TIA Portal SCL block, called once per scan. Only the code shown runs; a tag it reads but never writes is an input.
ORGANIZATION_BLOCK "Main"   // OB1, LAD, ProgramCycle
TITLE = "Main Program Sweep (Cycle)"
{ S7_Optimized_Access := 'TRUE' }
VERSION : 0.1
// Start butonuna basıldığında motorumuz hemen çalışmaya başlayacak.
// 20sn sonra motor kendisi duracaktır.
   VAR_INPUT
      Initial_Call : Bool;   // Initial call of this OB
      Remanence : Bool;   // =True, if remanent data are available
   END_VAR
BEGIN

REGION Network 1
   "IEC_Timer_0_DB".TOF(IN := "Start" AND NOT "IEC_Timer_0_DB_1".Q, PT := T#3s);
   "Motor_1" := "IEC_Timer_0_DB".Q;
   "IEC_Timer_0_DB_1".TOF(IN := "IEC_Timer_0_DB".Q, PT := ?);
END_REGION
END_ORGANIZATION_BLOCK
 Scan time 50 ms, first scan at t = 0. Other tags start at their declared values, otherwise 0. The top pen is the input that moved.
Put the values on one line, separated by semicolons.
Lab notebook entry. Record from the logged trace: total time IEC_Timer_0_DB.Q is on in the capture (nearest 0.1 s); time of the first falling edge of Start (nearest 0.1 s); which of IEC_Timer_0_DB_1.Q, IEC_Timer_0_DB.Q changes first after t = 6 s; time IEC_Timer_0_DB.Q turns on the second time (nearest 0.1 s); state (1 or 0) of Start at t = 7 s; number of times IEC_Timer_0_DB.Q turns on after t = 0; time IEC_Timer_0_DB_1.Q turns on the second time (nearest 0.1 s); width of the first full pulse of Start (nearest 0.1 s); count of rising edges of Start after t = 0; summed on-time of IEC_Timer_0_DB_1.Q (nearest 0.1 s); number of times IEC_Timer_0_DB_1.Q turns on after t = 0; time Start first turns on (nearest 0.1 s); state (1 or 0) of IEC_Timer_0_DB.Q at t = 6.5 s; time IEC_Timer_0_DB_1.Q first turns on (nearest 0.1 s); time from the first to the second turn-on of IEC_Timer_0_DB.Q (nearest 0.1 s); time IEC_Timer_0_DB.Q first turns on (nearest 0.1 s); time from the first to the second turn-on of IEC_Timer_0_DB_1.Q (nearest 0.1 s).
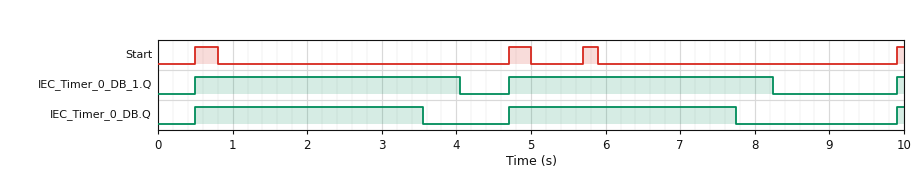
6.2 s; 0.8 s; IEC_Timer_0_DB.Q; 4.7 s; 0; 3; 4.7 s; 0.3 s; 4; 7.2 s; 3; 0.5 s; 1; 0.5 s; 4.2 s; 0.5 s; 4.2 s
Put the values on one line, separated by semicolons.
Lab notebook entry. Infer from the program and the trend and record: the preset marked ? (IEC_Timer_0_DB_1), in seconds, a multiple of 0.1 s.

0.5 s
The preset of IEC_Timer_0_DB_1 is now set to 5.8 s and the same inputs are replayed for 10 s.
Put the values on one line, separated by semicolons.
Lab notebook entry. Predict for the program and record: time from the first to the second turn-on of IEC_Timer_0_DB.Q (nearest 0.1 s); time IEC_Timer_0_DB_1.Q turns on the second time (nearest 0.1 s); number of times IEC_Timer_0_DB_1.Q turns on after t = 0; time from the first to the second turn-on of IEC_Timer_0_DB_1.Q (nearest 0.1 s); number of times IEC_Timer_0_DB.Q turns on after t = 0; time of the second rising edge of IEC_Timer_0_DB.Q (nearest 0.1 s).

9.4 s; 9.9 s; 2; 9.4 s; 2; 9.9 s
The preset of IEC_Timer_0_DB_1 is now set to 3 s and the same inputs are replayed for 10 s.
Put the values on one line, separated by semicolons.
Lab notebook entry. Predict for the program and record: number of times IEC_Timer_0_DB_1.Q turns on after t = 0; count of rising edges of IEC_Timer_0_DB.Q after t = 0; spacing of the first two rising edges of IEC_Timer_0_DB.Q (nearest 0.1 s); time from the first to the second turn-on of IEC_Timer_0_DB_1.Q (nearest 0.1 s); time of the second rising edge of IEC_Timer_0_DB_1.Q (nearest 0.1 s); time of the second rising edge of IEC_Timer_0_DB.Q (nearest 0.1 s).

2; 2; 9.4 s; 9.4 s; 9.9 s; 9.9 s
